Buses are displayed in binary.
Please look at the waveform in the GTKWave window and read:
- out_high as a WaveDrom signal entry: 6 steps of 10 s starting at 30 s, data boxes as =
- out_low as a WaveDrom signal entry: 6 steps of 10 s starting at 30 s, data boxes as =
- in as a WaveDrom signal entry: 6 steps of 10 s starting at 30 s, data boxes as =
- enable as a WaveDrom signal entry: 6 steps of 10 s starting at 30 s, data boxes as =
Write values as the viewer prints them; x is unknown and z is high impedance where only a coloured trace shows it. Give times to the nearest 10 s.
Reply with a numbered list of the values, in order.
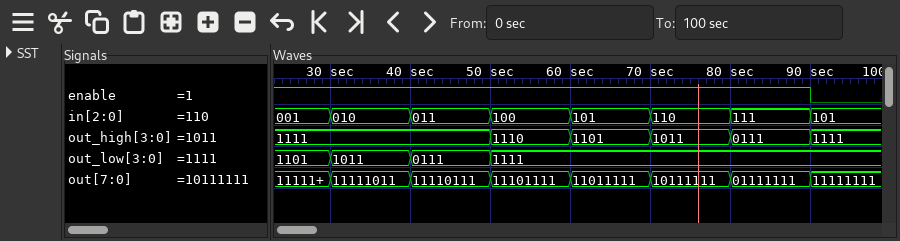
1. {name: 'out_high', wave: '=.====', data: '1111 1110 1101 1011 0111'}
2. {name: 'out_low', wave: '===...', data: '1011 0111 1111'}
3. {name: 'in', wave: '======', data: '010 011 100 101 110 111'}
4. {name: 'enable', wave: '1.....'}
